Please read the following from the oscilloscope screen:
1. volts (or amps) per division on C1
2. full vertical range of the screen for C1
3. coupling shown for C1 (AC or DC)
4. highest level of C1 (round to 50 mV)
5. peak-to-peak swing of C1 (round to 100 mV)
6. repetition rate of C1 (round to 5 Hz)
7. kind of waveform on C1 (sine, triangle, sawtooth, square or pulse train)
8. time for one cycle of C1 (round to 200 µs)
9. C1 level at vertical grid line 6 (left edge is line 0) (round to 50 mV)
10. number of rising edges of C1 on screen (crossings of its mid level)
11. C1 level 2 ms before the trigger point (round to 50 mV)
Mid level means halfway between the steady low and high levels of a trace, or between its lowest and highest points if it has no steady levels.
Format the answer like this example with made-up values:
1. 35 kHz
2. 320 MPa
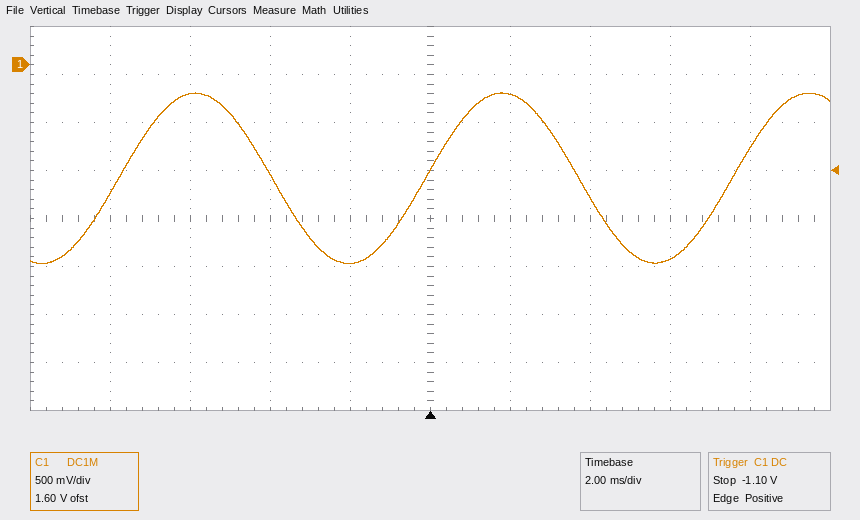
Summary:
1. 500 mV
2. 4 V
3. DC
4. -300 mV
5. 1.80 V
6. 130 Hz
7. sine
8. 7.6 ms
9. -300 mV
10. 3
11. -2.05 V
